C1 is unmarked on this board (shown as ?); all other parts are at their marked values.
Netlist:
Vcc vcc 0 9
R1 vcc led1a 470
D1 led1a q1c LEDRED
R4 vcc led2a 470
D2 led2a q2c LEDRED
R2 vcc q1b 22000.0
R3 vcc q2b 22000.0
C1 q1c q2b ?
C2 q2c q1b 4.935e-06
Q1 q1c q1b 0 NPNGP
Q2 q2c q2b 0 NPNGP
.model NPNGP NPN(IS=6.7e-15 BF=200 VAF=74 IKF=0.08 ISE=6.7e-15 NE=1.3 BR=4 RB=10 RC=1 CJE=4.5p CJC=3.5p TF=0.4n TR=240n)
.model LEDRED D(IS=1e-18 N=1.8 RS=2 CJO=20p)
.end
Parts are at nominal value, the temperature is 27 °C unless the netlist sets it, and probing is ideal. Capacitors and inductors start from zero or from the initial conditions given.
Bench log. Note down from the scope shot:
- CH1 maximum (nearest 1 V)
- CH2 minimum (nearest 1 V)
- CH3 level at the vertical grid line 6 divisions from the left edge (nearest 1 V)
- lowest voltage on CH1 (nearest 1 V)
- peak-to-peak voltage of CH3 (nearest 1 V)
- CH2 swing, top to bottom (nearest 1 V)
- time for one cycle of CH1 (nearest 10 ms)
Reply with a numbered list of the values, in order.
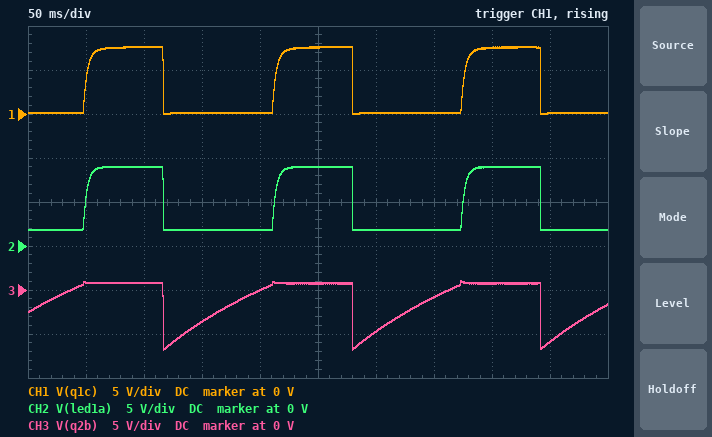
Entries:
1. 8 V
2. 2 V
3. -5 V
4. 0 V
5. 8 V
6. 7 V
7. 160 ms
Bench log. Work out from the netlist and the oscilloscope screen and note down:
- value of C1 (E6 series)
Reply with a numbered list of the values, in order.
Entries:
1. 6.8 µF
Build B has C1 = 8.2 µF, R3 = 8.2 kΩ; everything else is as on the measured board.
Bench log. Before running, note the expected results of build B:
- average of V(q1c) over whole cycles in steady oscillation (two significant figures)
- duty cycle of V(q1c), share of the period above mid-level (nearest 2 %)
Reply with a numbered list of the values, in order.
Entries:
1. 4.4 V
2. 60 %
